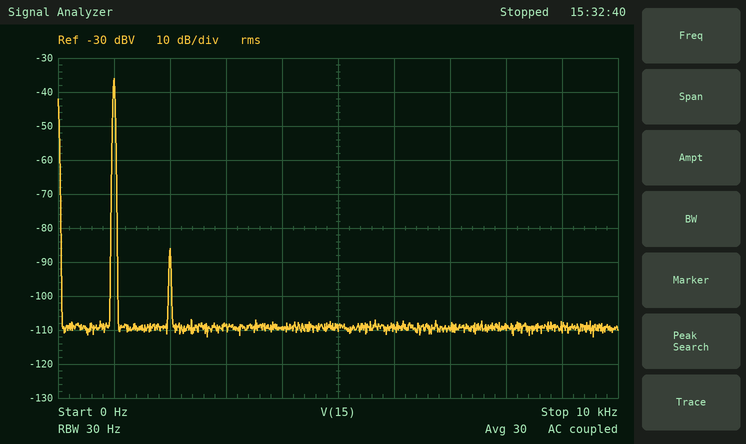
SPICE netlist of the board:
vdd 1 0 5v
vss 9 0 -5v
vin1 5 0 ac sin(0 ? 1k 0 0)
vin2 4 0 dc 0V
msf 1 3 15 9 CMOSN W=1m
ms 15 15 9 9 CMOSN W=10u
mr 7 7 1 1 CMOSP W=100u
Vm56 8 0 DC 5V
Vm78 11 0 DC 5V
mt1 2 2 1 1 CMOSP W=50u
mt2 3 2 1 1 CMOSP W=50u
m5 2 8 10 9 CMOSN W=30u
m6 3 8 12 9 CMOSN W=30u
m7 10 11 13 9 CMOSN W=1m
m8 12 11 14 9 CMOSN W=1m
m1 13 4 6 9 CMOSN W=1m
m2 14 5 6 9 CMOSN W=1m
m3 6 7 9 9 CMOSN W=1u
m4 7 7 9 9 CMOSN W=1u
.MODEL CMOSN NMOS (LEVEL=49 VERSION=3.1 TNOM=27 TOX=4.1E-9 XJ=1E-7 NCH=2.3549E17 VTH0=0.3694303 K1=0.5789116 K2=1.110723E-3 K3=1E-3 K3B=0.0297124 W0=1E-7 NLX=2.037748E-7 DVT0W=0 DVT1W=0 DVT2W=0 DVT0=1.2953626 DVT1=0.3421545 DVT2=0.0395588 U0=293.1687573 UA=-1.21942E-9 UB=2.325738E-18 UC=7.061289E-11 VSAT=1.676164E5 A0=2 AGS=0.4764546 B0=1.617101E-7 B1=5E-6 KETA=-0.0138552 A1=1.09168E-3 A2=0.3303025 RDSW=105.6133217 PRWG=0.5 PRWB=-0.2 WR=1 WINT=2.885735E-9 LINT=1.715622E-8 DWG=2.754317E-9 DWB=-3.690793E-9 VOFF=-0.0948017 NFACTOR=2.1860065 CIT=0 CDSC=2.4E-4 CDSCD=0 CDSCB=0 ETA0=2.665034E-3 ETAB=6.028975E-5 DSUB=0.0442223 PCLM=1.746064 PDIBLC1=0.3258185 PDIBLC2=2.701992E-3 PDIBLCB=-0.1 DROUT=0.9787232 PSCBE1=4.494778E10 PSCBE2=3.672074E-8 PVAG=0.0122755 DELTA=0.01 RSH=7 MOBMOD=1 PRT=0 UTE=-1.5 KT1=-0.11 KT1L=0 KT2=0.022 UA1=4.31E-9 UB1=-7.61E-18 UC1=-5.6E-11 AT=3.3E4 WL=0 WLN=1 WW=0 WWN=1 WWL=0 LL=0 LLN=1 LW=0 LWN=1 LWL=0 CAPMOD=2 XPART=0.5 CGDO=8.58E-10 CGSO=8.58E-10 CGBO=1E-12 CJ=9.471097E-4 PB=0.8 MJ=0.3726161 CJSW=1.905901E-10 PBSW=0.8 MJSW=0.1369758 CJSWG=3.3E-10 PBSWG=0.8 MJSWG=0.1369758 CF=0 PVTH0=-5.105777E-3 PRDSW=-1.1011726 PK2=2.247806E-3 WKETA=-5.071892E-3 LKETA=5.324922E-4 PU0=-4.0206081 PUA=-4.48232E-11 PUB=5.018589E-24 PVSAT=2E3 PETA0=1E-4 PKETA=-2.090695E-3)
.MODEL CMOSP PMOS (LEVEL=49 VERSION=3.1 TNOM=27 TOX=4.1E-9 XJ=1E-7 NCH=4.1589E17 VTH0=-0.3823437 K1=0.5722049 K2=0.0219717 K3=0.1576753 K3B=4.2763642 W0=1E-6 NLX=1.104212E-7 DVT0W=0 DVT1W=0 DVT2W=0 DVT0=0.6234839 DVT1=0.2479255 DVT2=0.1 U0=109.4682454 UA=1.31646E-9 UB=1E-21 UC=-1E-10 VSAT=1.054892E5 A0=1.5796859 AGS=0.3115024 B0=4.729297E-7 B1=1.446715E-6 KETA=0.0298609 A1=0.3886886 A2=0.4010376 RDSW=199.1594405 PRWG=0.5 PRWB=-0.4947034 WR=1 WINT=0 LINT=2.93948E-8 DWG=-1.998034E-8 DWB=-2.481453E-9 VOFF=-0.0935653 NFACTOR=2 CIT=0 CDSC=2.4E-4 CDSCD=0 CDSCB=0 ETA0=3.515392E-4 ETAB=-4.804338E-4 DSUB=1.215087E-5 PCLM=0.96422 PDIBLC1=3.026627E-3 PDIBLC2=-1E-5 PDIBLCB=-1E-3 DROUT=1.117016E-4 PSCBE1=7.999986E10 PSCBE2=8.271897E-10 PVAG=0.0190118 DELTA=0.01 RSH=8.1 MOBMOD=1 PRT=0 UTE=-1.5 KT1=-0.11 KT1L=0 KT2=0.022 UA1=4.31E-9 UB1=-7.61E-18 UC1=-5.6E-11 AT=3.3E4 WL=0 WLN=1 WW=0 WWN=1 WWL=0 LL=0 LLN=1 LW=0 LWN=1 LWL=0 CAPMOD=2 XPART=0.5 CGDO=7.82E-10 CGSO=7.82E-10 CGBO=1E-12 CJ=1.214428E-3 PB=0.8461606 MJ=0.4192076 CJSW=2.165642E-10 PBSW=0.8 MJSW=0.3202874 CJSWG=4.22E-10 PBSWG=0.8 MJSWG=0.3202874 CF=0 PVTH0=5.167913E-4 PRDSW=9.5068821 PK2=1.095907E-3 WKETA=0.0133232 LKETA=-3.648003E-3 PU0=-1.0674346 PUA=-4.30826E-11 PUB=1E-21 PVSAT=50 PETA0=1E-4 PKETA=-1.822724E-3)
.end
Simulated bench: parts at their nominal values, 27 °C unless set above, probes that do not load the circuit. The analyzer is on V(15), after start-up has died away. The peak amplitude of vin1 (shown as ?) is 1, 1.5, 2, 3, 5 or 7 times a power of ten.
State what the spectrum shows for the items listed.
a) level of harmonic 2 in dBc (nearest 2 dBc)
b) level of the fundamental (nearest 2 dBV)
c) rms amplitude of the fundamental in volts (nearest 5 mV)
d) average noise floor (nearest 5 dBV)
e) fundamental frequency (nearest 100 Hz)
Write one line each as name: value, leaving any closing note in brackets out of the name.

level of harmonic 2 in dBc: -50 dBc
level of the fundamental: -36 dBV
rms amplitude of the fundamental in volts: 15 mV
average noise floor: -110 dBV
fundamental frequency: 1.0 kHz
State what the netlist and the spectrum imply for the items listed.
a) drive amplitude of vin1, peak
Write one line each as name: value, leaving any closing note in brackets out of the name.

drive amplitude of vin1, peak: 20 µV
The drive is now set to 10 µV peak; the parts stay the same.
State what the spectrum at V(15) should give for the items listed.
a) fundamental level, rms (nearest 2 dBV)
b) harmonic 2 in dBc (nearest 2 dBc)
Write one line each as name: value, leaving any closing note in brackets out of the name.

fundamental level, rms: -42 dBV
harmonic 2 in dBc: -56 dBc
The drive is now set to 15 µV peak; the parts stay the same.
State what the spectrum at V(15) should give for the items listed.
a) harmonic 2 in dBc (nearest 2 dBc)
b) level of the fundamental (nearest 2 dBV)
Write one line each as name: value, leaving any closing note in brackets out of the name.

harmonic 2 in dBc: -52 dBc
level of the fundamental: -38 dBV
